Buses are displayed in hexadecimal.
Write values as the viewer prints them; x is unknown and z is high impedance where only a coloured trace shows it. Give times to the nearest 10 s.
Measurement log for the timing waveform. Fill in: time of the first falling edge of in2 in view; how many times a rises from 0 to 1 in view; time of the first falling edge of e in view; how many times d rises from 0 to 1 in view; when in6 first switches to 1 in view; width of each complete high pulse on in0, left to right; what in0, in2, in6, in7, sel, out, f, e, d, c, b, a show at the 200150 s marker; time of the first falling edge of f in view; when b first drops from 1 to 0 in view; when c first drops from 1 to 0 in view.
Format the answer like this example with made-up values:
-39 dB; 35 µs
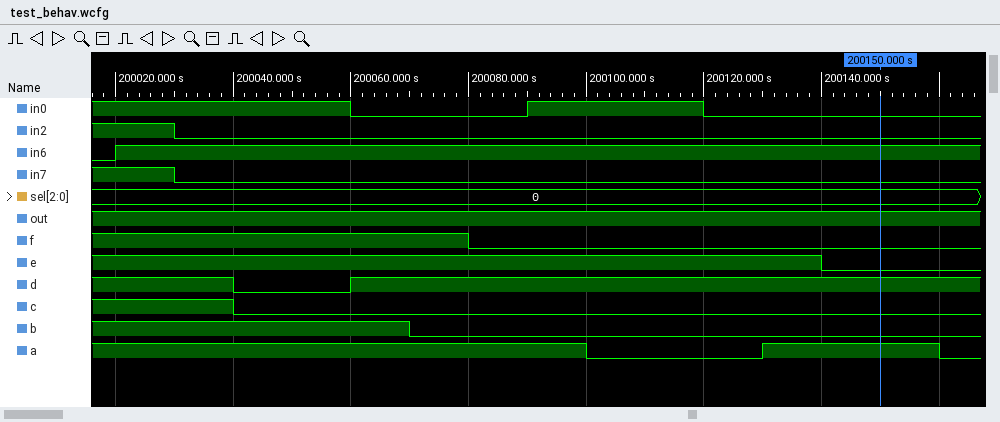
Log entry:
200030 s; 1; 200140 s; 1; 200020 s; 30 s; in0=0, in2=0, in6=1, in7=0, sel=0, out=1, f=0, e=0, d=1, c=0, b=0, a=1; 200080 s; 200070 s; 200040 s
